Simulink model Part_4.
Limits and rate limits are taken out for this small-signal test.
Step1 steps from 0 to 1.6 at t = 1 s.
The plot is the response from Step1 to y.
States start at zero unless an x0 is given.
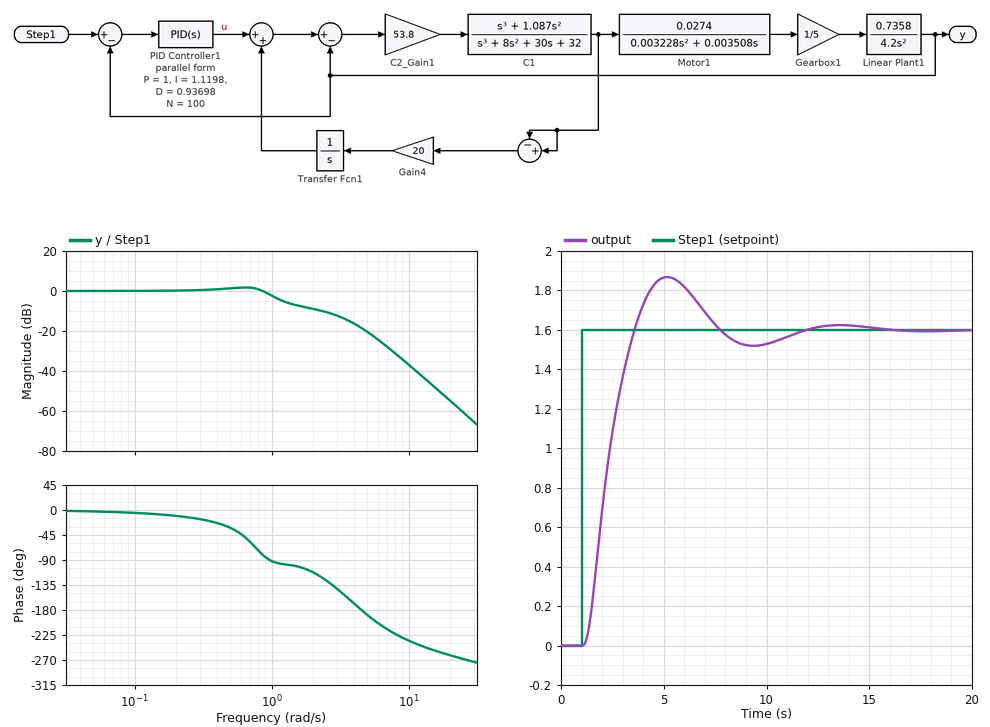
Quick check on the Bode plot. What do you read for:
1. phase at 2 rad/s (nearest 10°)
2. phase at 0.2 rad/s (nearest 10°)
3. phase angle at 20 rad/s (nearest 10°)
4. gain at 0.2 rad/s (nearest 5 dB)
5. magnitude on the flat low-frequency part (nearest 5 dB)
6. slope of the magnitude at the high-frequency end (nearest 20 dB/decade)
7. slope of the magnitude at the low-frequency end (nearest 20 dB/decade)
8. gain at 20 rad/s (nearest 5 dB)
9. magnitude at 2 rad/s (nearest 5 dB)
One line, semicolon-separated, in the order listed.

-110°; -10°; -260°; 0 dB; 0 dB; -60 dB/decade; 0 dB/decade; -55 dB; -10 dB
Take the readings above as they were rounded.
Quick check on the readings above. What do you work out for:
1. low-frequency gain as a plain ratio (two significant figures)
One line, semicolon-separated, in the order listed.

1.0
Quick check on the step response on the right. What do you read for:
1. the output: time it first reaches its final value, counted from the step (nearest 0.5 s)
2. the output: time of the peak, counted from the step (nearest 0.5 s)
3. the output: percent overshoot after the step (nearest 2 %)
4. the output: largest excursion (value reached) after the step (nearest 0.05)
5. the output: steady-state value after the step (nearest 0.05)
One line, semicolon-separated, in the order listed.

2.5 s; 4.0 s; 16 %; 1.85; 1.60
